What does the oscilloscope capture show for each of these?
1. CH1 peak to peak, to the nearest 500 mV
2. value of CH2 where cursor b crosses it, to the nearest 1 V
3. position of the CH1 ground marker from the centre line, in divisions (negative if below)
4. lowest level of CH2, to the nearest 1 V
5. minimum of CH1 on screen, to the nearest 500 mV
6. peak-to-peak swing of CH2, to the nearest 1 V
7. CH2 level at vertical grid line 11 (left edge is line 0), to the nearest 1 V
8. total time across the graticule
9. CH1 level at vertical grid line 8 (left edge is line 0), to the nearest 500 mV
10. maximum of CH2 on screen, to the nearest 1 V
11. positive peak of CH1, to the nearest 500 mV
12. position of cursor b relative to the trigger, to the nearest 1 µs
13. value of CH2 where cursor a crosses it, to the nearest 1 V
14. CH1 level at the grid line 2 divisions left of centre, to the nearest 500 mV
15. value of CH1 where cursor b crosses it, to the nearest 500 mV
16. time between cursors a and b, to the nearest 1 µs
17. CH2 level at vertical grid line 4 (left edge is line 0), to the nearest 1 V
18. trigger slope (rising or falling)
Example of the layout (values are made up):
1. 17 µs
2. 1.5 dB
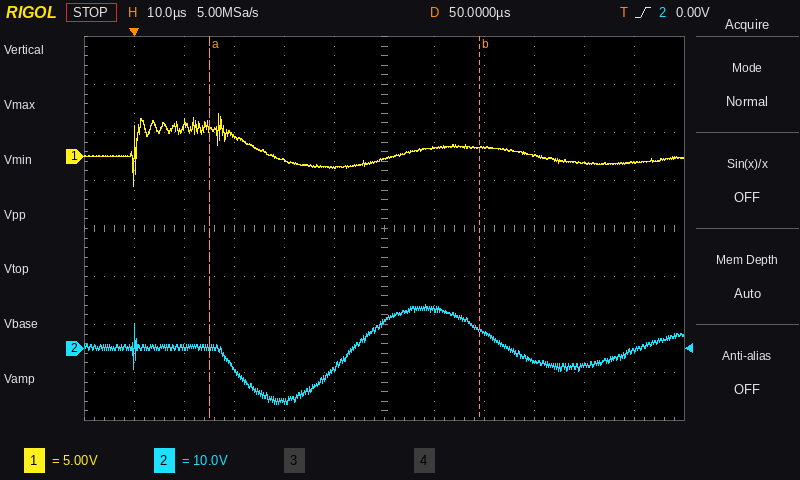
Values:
1. 7.5 V
2. 4 V
3. +1.5 div
4. -12 V
5. -3.0 V
6. 21 V
7. 0 V
8. 120 µs
9. 1.0 V
10. 9 V
11. 4.5 V
12. +69 µs
13. 0 V
14. -500 mV
15. 1.0 V
16. 54 µs
17. -11 V
18. rising
